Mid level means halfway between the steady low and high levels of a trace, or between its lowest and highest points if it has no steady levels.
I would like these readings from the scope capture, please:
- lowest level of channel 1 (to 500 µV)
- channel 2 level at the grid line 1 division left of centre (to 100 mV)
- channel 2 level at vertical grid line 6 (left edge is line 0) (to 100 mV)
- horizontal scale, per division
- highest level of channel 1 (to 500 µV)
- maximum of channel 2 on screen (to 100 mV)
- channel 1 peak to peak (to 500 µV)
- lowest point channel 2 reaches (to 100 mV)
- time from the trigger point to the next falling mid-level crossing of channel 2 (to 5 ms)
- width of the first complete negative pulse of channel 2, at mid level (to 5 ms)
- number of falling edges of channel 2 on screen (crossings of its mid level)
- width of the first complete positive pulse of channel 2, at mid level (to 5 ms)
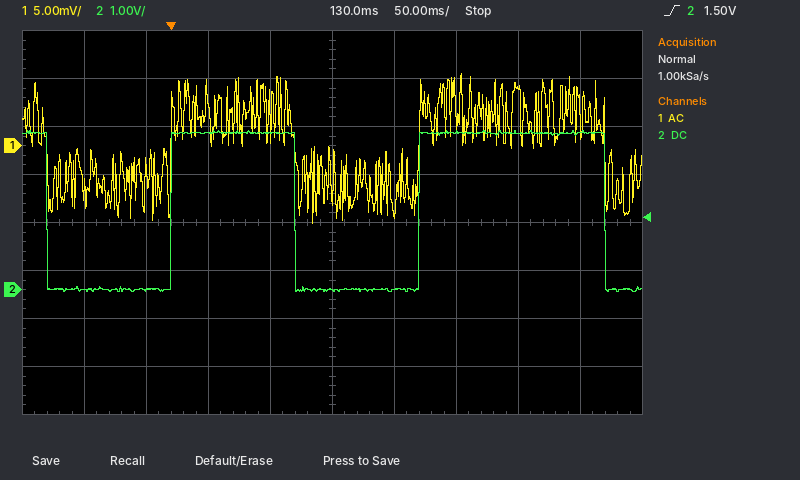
-8.0 mV
3.3 V
0.0 V
50 ms
7.5 mV
3.3 V
15.5 mV
0.0 V
100 ms
100 ms
3
100 ms
